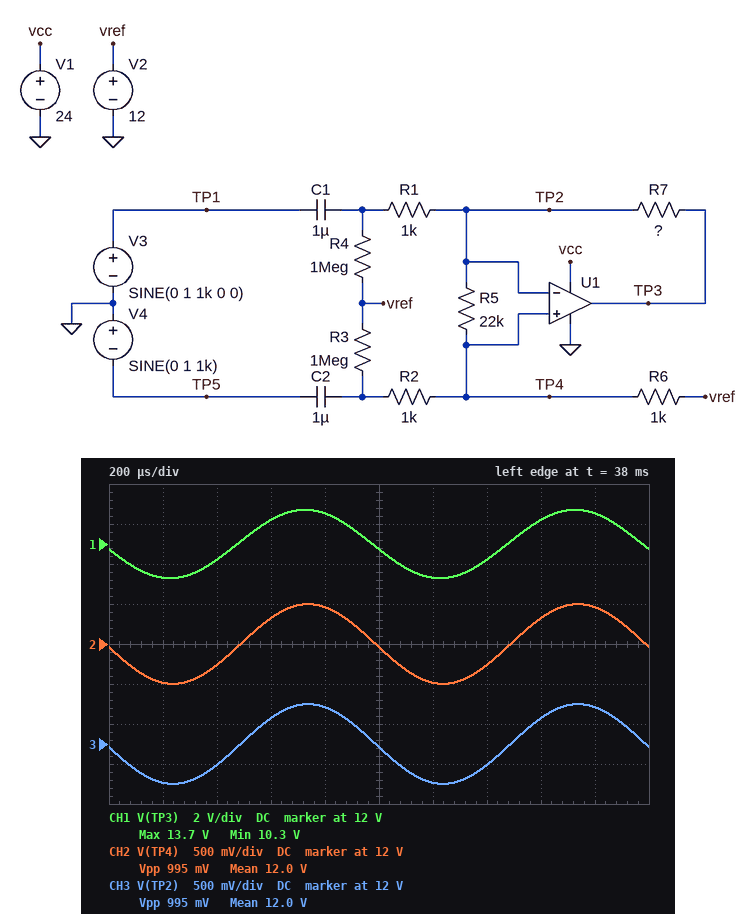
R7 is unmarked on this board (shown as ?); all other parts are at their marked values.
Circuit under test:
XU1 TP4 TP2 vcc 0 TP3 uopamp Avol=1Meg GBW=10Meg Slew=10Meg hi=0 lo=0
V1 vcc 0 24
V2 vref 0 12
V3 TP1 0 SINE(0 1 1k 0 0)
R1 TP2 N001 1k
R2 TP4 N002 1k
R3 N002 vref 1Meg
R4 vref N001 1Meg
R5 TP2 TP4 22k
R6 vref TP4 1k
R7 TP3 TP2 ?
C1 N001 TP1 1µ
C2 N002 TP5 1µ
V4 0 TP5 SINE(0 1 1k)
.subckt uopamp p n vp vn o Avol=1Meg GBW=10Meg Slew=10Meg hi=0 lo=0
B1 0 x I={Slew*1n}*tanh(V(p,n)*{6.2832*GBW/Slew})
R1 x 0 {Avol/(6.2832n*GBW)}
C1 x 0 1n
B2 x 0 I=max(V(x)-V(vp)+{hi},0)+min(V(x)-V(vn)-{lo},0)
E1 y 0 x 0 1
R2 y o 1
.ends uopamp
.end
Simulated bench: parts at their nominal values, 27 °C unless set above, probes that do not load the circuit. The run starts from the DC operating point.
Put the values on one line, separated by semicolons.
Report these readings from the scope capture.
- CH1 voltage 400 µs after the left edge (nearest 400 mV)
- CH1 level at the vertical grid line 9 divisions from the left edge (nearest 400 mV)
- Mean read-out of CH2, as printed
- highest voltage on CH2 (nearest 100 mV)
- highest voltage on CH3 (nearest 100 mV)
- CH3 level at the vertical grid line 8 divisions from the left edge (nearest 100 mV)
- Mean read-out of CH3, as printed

11.2 V; 13.6 V; 12.0 V; 12.5 V; 12.5 V; 12.3 V; 12.0 V
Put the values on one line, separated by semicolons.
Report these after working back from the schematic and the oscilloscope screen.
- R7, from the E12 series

820 Ω
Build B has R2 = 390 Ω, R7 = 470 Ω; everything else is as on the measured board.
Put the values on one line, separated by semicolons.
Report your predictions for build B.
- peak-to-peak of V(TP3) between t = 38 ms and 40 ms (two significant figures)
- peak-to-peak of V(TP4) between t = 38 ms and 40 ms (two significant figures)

3.0 V; 1.4 V
